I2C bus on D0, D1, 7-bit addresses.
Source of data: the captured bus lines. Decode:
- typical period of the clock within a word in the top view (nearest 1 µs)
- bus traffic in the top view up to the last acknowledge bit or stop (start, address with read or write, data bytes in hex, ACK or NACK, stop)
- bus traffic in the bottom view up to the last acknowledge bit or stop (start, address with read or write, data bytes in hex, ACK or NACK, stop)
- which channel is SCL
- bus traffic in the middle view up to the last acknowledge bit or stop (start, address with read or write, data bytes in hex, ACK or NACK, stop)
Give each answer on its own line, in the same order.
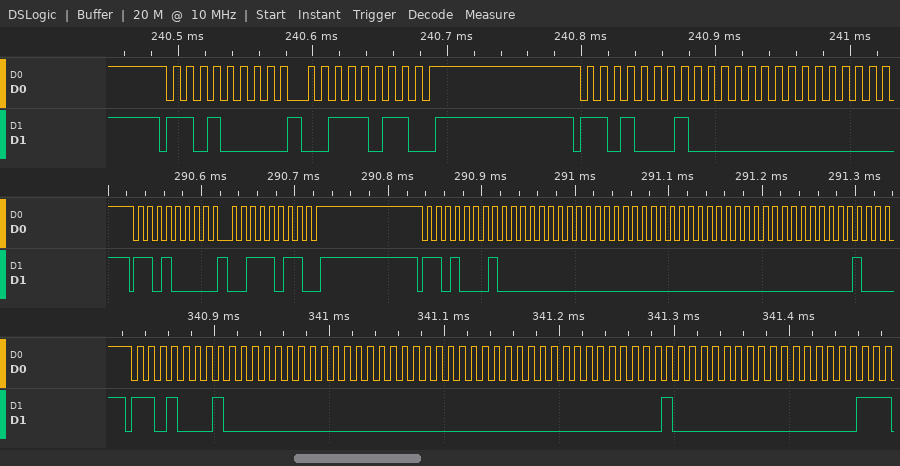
10 µs
start, address 68 write ACK, 3B ACK, stop, start, address 68 read ACK, 00 ACK
start, address 68 read ACK, 00 ACK, 00 ACK, 00 ACK, 00 ACK, 40 ACK, 00 ACK
D0
start, address 68 write ACK, 3B ACK, stop, start, address 68 read ACK, 00 ACK, 00 ACK, 00 ACK, 00 ACK
